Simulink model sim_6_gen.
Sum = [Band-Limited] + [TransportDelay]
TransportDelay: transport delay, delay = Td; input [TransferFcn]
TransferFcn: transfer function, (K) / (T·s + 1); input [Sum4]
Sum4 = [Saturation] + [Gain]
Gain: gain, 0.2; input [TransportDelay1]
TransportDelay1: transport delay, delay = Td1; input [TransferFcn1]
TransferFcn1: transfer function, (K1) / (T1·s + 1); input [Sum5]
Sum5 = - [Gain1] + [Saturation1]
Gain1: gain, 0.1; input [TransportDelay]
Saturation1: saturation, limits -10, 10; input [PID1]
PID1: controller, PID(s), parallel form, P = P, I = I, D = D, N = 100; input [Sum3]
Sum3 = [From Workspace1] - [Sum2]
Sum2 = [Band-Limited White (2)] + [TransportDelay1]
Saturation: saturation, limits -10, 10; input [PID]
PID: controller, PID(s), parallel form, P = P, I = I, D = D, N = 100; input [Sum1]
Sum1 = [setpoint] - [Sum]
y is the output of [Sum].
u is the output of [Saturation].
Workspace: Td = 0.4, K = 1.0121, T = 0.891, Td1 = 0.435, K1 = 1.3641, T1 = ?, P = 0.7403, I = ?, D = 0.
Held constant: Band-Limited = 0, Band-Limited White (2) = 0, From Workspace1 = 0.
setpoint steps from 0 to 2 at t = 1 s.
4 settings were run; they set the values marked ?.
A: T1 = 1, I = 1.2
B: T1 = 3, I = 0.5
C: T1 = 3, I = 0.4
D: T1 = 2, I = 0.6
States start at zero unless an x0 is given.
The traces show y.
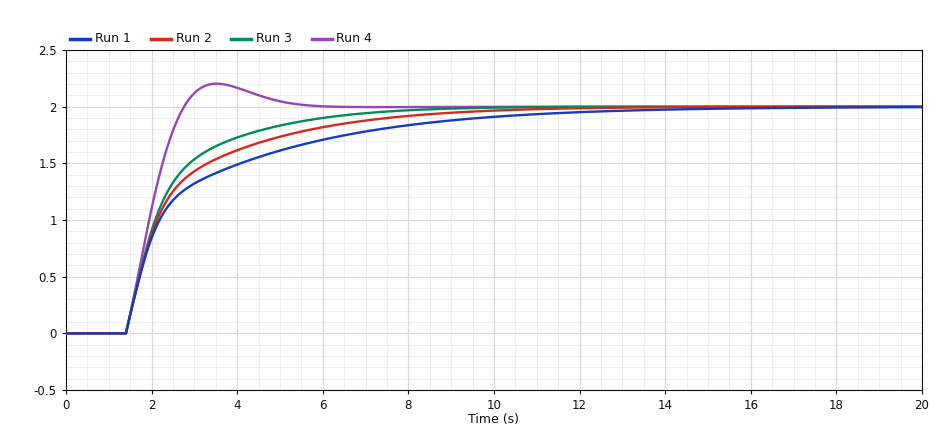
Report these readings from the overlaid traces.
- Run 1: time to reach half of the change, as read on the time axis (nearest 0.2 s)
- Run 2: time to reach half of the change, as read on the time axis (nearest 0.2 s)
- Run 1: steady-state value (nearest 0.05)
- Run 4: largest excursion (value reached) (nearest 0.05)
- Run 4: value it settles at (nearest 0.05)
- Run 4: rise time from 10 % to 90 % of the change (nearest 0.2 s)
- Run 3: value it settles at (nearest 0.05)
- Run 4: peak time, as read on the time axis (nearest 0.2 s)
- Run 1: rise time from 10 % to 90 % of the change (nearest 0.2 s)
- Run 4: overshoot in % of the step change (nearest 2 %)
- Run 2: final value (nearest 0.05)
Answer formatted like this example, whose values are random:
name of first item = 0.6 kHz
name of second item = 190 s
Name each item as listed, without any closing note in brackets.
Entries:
Run 1: time to reach half of the change, as read on the time axis = 2.2 s
Run 2: time to reach half of the change, as read on the time axis = 2.2 s
Run 1: steady-state value = 2.00
Run 4: largest excursion (value reached) = 2.20
Run 4: value it settles at = 2.00
Run 4: rise time from 10 % to 90 % of the change = 1.0 s
Run 3: value it settles at = 2.00
Run 4: peak time, as read on the time axis = 3.6 s
Run 1: rise time from 10 % to 90 % of the change = 5.8 s
Run 4: overshoot in % of the step change = 10 %
Run 2: final value = 2.00
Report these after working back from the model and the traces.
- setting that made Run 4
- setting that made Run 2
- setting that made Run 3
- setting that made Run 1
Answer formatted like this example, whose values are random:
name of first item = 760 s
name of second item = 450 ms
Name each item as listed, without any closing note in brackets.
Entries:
setting that made Run 4 = A
setting that made Run 2 = B
setting that made Run 3 = D
setting that made Run 1 = C
